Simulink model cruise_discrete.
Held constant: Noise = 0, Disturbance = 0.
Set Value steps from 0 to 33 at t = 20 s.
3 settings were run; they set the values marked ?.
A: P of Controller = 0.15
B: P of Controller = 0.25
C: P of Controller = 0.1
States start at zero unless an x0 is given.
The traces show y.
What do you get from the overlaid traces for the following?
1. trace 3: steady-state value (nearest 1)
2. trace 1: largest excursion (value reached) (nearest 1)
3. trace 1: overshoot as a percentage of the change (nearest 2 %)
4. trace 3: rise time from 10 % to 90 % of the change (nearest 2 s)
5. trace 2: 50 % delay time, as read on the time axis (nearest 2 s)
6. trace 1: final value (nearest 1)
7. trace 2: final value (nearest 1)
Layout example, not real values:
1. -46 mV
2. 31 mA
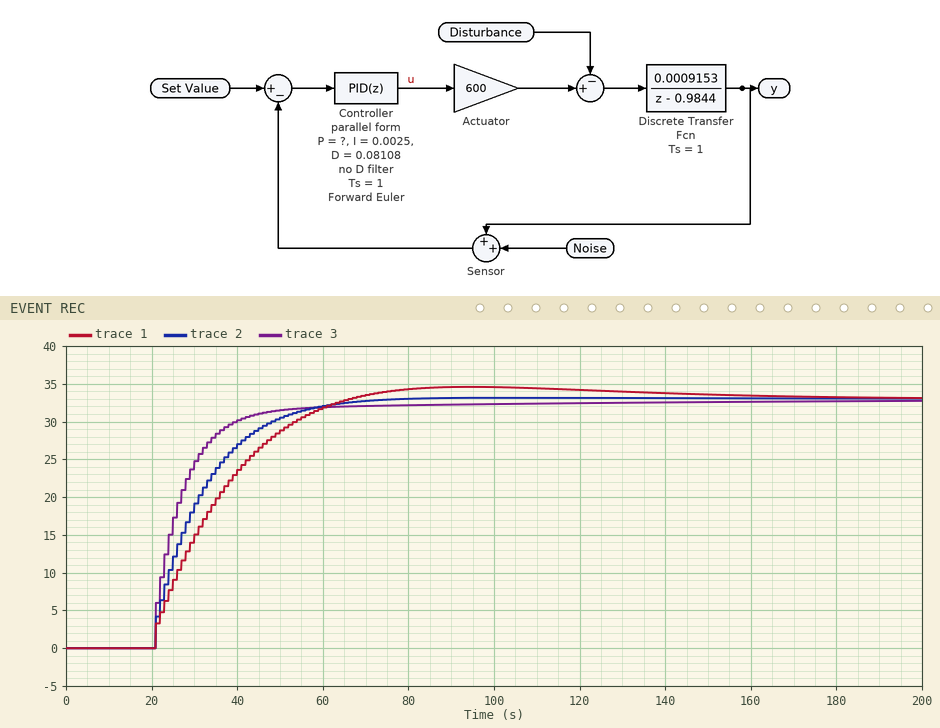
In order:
1. 33
2. 35
3. 4 %
4. 18 s
5. 28 s
6. 33
7. 33
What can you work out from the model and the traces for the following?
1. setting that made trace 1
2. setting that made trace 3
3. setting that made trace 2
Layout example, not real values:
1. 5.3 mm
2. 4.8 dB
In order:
1. C
2. B
3. A
